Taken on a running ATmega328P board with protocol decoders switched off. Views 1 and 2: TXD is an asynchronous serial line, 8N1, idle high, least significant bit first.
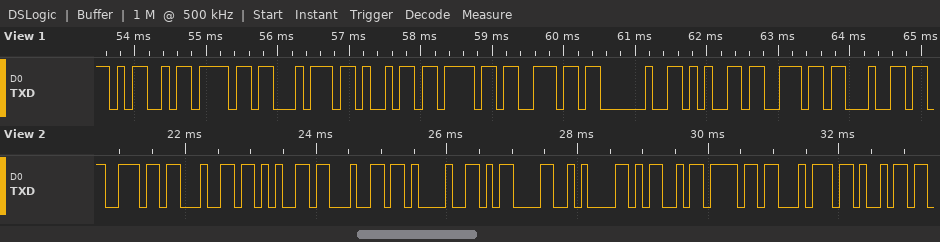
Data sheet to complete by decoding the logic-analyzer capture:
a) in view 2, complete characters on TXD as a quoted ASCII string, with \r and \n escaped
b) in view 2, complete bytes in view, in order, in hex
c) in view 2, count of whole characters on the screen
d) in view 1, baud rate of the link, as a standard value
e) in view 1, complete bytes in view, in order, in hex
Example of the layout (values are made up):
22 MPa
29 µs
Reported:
"nded!\r\nMoti"
6E 64 65 64 21 0D 0A 4D 6F 74 69
11
9600 baud
4D 6F 74 69 6F 6E 20 65 6E 64
